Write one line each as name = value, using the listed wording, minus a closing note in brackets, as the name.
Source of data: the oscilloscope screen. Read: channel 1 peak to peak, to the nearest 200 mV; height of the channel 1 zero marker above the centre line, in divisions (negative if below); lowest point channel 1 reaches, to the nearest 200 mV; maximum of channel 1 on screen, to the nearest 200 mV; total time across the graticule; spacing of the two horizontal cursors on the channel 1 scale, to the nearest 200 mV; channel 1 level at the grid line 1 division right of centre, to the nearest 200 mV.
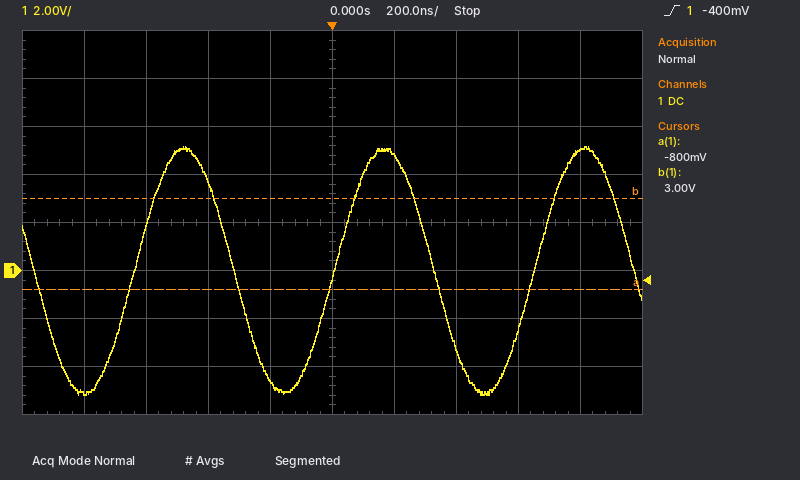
channel 1 peak to peak, to the nearest 200 mV = 10.4 V
height of the channel 1 zero marker above the centre line, in divisions = -1.0 div
lowest point channel 1 reaches, to the nearest 200 mV = -5.2 V
maximum of channel 1 on screen, to the nearest 200 mV = 5.2 V
total time across the graticule = 2 µs
spacing of the two horizontal cursors on the channel 1 scale, to the nearest 200 mV = 3.8 V
channel 1 level at the grid line 1 division right of centre, to the nearest 200 mV = 4.8 V
